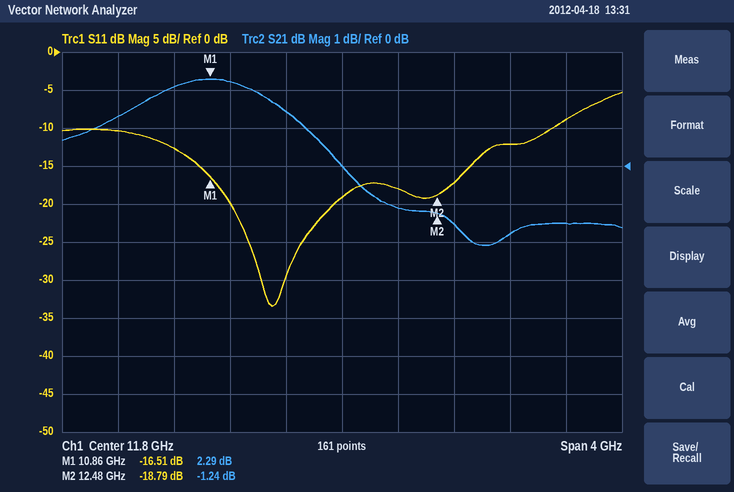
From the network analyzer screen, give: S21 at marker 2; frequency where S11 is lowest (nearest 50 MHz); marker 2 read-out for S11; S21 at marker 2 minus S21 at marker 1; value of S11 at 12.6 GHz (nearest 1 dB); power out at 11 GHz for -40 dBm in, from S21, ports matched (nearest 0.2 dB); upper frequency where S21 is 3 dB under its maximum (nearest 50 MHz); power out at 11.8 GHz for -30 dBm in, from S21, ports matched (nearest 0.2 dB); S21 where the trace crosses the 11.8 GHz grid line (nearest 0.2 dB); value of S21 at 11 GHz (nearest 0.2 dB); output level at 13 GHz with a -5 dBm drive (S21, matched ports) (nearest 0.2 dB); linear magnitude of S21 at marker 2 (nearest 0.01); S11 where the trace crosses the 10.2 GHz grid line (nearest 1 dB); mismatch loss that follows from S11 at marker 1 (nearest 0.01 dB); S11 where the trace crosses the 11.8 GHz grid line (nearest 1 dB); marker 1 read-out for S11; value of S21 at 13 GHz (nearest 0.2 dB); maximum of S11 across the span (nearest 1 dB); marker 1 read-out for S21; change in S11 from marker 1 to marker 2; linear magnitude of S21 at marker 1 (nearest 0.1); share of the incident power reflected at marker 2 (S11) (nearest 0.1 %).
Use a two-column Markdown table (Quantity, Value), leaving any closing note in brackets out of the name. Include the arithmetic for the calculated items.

| Quantity | Value |
|---|---|
| S21 at marker 2 | -1.24 dB |
| frequency where S11 is lowest | 11.30 GHz |
| marker 2 read-out for S11 | -18.79 dB |
| S21 at marker 2 minus S21 at marker 1 | -1.24 − (2.29) = -3.53 dB |
| value of S11 at 12.6 GHz | -17 dB |
| power out at 11 GHz for -40 dBm in, from S21, ports matched | -40 dBm + (2.2 dB) = -37.8 dBm |
| upper frequency where S21 is 3 dB under its maximum | 12.00 GHz |
| power out at 11.8 GHz for -30 dBm in, from S21, ports matched | -30 dBm + (0.0 dB) = -30.0 dBm |
| S21 where the trace crosses the 11.8 GHz grid line | 0.0 dB |
| value of S21 at 11 GHz | 2.2 dB |
| output level at 13 GHz with a -5 dBm drive (S21, matched ports) | -5 dBm + (-1.8 dB) = -6.8 dBm |
| linear magnitude of S21 at marker 2 | 10^(-1.24/20) ≈ 0.87 |
| S11 where the trace crosses the 10.2 GHz grid line | -10 dB |
| mismatch loss that follows from S11 at marker 1 | −10 log10(1 − 10^(-16.51/10)) ≈ 0.10 dB |
| S11 where the trace crosses the 11.8 GHz grid line | -19 dB |
| marker 1 read-out for S11 | -16.51 dB |
| value of S21 at 13 GHz | -1.8 dB |
| maximum of S11 across the span | -5 dB |
| marker 1 read-out for S21 | 2.29 dB |
| change in S11 from marker 1 to marker 2 | -18.79 − (-16.51) = -2.28 dB |
| linear magnitude of S21 at marker 1 | 10^(2.29/20) ≈ 1.3 |
| share of the incident power reflected at marker 2 (S11) | 10^(-18.79/10) ≈ 1.3 % |
